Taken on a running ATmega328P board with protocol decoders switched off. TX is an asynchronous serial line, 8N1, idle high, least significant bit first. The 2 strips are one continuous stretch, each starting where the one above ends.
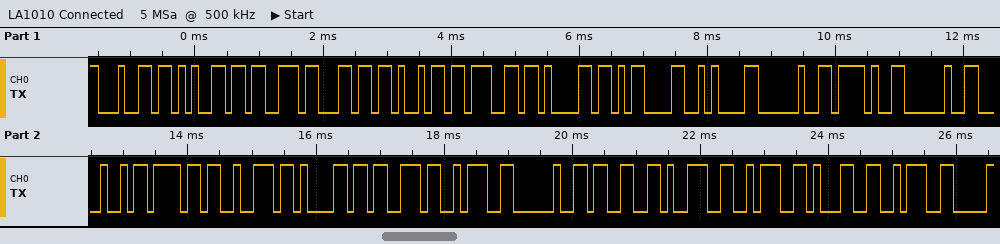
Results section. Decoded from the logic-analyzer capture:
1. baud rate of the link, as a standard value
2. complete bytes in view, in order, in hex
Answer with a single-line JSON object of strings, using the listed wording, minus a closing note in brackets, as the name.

{"baud rate of the link, as a standard value": "9600 baud", "complete bytes in view, in order, in hex": "64 65 73 6C 69 67 61 0D 0A 20 2F 20 48 6F 72 61 73 3A 20 33 39 3A 31 3A"}
